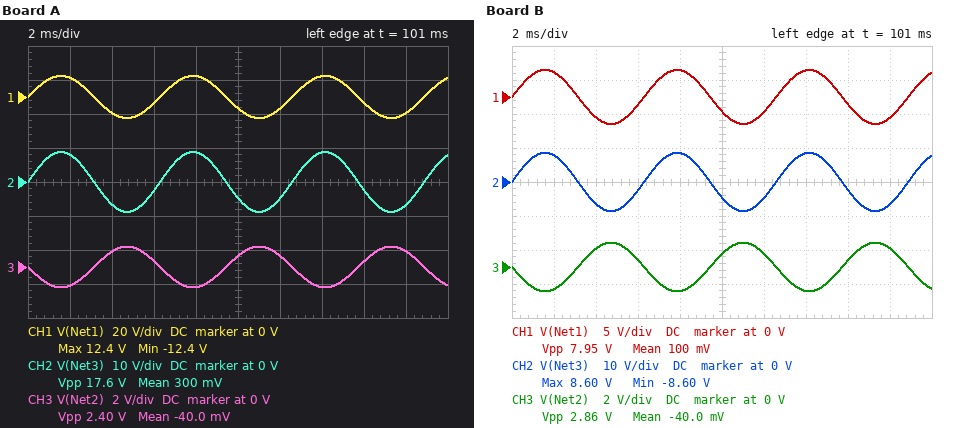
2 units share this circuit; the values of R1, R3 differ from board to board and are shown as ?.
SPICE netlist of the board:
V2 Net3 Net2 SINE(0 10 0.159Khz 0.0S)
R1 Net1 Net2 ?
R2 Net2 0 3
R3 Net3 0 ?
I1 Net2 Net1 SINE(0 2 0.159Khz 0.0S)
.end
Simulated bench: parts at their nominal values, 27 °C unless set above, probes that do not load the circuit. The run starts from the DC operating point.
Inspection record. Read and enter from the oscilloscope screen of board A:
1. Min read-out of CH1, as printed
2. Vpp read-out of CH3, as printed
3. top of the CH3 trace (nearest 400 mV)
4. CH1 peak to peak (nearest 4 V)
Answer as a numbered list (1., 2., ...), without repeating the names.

1. -12.4 V
2. 2.40 V
3. 1.2 V
4. 24 V
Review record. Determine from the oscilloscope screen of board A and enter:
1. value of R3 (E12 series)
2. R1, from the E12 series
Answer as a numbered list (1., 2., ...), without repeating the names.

1. 22 Ω
2. 6.8 Ω
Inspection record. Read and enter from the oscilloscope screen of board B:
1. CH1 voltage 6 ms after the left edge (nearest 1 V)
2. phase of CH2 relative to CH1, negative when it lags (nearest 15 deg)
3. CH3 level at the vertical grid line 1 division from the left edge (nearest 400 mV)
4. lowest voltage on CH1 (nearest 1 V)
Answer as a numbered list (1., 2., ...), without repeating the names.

1. -1 V
2. 0 deg
3. -1.2 V
4. -4 V
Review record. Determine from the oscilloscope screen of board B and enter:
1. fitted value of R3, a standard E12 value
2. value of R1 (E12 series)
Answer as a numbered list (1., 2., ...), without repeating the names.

1. 18 Ω
2. 2.7 Ω
